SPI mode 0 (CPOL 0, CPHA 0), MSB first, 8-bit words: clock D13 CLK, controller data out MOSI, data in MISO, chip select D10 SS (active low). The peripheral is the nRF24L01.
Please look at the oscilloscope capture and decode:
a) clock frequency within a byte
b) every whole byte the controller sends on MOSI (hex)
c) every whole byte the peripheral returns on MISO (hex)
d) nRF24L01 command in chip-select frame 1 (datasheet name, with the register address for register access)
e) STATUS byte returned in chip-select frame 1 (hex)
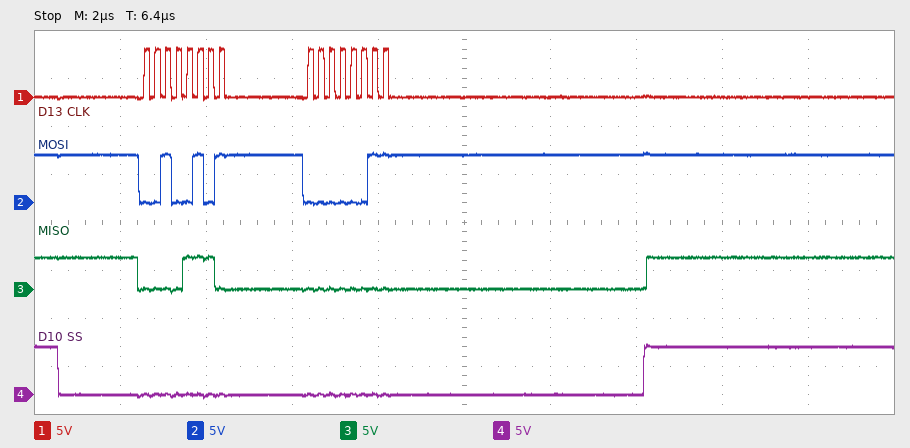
4 MHz
25 03
0E 00
W_REGISTER 0x05
0x0E
